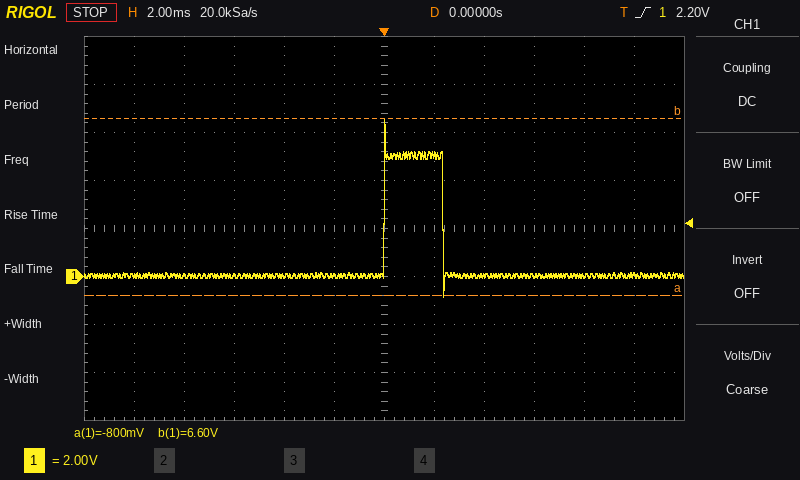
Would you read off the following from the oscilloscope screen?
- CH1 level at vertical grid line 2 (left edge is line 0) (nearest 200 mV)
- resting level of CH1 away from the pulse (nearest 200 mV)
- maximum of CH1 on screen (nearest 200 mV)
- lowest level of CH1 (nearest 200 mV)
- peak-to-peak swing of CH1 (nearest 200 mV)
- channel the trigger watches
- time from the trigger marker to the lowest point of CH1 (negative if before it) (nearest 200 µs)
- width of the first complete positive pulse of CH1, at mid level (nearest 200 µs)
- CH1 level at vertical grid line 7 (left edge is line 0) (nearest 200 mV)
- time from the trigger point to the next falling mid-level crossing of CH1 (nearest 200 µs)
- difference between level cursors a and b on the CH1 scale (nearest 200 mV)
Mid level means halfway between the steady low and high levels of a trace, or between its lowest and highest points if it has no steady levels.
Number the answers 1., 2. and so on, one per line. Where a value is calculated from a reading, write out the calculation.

1. 0.0 V
2. 0.0 V
3. 6.6 V
4. -800 mV
5. 6.6 V − (-800 mV) = 7.4 V
6. CH1
7. +2.4 ms
8. 2.4 ms
9. 5.0 V
10. 2.4 ms
11. 7.4 V
